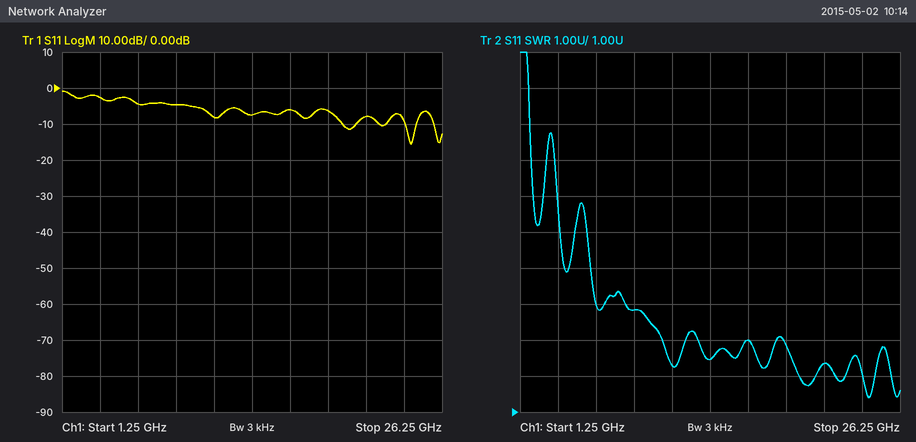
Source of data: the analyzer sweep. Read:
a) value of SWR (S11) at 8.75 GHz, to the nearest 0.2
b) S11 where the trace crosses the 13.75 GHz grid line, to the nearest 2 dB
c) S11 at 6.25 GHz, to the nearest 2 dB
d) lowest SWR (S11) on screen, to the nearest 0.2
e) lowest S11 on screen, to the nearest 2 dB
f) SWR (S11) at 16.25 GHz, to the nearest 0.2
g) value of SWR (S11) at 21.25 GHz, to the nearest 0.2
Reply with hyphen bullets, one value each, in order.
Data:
- 3.8
- -8 dB
- -4 dB
- 1.4
- -16 dB
- 3.0
- 2.4
